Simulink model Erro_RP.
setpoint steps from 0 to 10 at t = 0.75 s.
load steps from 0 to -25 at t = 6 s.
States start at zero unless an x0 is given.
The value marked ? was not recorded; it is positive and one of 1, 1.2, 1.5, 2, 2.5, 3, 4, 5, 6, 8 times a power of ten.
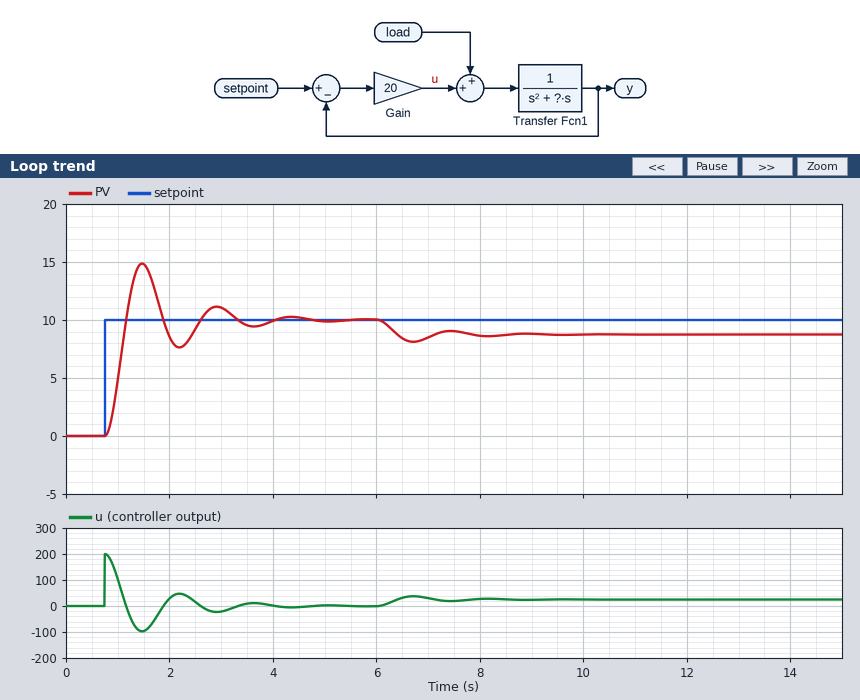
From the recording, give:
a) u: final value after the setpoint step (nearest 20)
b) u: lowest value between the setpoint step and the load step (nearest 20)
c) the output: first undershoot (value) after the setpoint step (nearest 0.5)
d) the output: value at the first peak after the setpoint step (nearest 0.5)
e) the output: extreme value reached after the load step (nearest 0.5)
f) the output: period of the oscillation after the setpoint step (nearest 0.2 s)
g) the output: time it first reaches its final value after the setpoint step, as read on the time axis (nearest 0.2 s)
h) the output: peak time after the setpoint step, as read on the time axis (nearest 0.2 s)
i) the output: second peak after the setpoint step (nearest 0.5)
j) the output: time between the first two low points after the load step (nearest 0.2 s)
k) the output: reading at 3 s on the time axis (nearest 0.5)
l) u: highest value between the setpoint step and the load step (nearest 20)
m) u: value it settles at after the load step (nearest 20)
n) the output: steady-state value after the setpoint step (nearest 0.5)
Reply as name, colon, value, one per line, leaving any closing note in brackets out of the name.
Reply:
u: final value after the setpoint step: 0
u: lowest value between the setpoint step and the load step: -100
the output: first undershoot (value) after the setpoint step: 7.5
the output: value at the first peak after the setpoint step: 15.0
the output: extreme value reached after the load step: 8.0
the output: period of the oscillation after the setpoint step: 1.4 s
the output: time it first reaches its final value after the setpoint step, as read on the time axis: 1.2 s
the output: peak time after the setpoint step, as read on the time axis: 1.4 s
the output: second peak after the setpoint step: 11.0
the output: time between the first two low points after the load step: 1.4 s
the output: reading at 3 s on the time axis: 11.0
u: highest value between the setpoint step and the load step: 200
u: value it settles at after the load step: 20
the output: steady-state value after the setpoint step: 10.0
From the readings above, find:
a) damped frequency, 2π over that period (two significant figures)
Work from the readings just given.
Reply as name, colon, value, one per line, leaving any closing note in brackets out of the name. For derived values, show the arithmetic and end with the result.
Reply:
damped frequency, 2π over that period: 2π / 1.4 = 4.5 rad/s
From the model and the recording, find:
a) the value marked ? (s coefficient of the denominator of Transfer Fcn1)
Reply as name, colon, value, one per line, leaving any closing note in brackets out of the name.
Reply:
the value marked ?: 2
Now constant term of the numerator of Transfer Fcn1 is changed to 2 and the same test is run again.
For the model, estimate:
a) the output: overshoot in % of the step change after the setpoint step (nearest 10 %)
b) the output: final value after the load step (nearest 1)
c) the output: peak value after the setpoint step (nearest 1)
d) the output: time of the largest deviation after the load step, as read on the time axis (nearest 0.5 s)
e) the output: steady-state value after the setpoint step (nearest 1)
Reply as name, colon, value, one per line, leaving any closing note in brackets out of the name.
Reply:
the output: overshoot in % of the step change after the setpoint step: 60 %
the output: final value after the load step: 9
the output: peak value after the setpoint step: 16
the output: time of the largest deviation after the load step, as read on the time axis: 6.5 s
the output: steady-state value after the setpoint step: 10
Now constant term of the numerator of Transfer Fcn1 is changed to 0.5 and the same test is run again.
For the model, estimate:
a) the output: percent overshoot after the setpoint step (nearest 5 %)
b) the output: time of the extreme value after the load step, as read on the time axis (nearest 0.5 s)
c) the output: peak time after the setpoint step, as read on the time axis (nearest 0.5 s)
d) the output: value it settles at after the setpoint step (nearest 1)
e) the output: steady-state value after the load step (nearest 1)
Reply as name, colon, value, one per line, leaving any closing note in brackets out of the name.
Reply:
the output: percent overshoot after the setpoint step: 35 %
the output: time of the extreme value after the load step, as read on the time axis: 7.0 s
the output: peak time after the setpoint step, as read on the time axis: 2.0 s
the output: value it settles at after the setpoint step: 10
the output: steady-state value after the load step: 9
